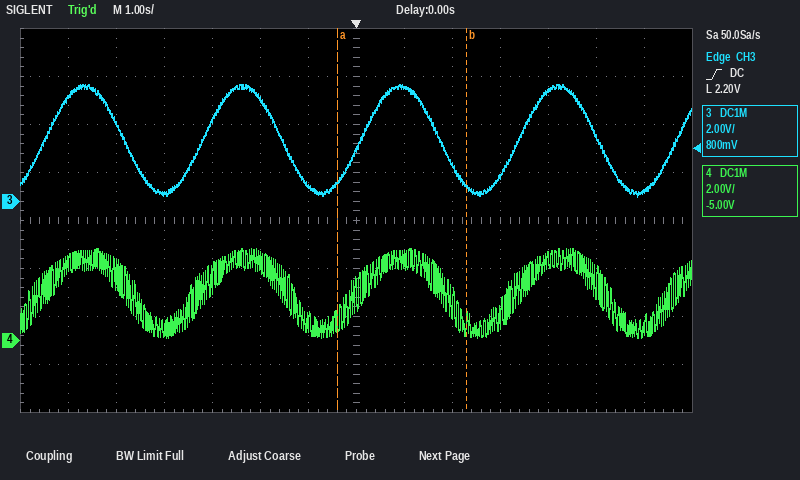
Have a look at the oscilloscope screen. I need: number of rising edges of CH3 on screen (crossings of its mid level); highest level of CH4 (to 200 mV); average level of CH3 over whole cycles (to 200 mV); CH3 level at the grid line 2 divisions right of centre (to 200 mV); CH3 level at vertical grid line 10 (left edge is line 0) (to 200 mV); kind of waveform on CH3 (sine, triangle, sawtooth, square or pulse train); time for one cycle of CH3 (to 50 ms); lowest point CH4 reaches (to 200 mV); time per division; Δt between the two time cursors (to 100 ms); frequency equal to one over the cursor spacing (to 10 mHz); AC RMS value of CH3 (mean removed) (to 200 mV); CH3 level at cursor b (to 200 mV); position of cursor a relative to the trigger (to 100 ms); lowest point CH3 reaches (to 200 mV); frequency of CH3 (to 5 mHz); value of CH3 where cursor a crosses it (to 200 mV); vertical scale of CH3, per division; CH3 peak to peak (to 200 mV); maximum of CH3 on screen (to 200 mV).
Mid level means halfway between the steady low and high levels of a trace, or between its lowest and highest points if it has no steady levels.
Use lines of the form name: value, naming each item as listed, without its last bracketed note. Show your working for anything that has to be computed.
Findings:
number of rising edges of CH3 on screen: 5
highest level of CH4: 3.8 V
average level of CH3 over whole cycles: (4.8 V + (200 mV)) / 2 ≈ 2.50 V, so 2.6 V to the nearest 200 mV
CH3 level at the grid line 2 divisions right of centre: 1.6 V
CH3 level at vertical grid line 10 (left edge is line 0): 1.0 V
kind of waveform on CH3: sine
time for one cycle of CH3: 3.30 s
lowest point CH4 reaches: 200 mV
time per division: 1 s
Δt between the two time cursors: 2.7 s
frequency equal to one over the cursor spacing: 1 / 2.7 s ≈ 370 mHz
AC RMS value of CH3 (mean removed): 4.6 V / (2√2) ≈ 1.6 V
CH3 level at cursor b: 600 mV
position of cursor a relative to the trigger: -400 ms
lowest point CH3 reaches: 200 mV
frequency of CH3: 1 / 3.30 s ≈ 303 mHz, so 305 mHz to the nearest 5 mHz
value of CH3 where cursor a crosses it: 800 mV
vertical scale of CH3, per division: 2 V
CH3 peak to peak: 4.8 V − (200 mV) = 4.6 V
maximum of CH3 on screen: 4.8 V
